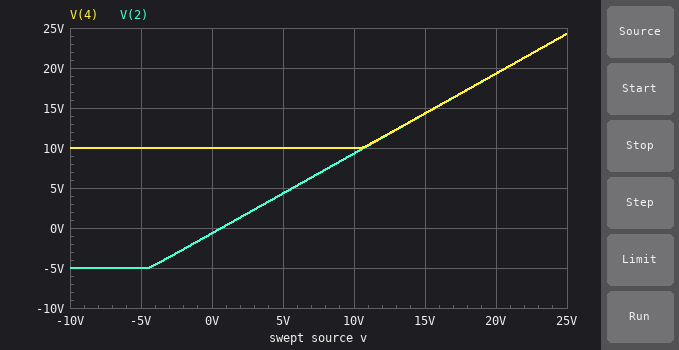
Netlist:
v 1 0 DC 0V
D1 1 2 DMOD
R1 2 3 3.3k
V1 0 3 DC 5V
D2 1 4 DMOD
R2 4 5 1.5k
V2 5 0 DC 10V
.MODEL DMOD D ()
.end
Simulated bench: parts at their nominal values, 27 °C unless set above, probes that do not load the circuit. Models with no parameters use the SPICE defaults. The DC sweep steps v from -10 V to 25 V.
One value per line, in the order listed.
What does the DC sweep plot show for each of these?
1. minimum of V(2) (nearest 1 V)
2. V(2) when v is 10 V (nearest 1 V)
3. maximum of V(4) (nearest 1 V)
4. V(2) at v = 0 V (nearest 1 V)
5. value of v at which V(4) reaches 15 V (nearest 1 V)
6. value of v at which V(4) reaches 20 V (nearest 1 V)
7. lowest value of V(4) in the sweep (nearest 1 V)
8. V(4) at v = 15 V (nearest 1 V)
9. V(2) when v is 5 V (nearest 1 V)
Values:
-5 V
9 V
24 V
-1 V
16 V
21 V
10 V
14 V
4 V
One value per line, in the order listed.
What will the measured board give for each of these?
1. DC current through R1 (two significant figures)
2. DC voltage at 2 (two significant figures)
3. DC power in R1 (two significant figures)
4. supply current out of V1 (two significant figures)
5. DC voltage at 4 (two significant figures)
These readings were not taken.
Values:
1.3 mA
-660 mV
5.7 mW
1.3 mA
10 V
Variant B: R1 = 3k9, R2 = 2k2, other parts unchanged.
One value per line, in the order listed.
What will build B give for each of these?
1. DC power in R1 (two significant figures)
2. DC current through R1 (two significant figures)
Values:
4.8 mW
1.1 mA
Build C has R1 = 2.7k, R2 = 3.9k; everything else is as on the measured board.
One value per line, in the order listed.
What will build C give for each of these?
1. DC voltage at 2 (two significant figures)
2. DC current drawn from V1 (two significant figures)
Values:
-670 mV
1.6 mA
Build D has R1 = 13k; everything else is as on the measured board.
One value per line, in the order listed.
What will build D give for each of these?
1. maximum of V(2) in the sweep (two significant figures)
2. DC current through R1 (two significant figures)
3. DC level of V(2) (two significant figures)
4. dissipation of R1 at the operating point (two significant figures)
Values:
24 V
340 µA
-630 mV
1.5 mW
